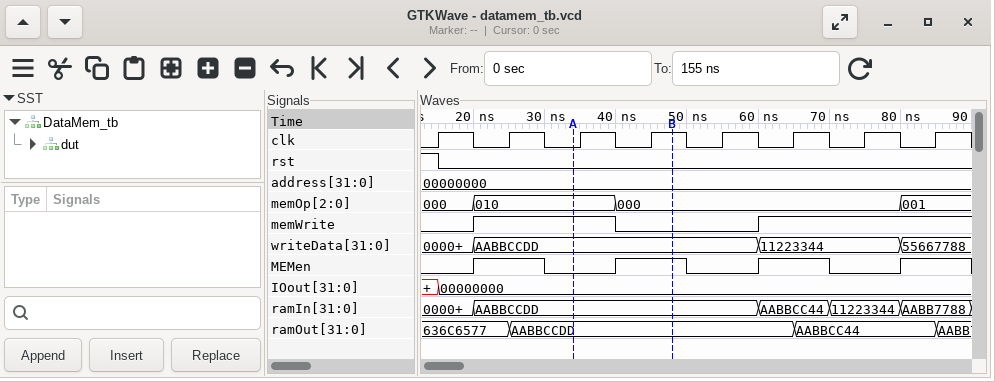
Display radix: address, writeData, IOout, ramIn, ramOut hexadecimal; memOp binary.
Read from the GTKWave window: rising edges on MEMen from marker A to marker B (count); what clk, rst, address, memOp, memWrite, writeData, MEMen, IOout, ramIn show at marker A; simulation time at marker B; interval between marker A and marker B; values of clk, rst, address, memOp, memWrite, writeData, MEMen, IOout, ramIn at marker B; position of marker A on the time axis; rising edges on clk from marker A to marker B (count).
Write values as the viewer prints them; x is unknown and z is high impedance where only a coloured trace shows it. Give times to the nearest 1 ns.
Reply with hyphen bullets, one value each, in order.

- 1
- clk=0, rst=0, address=00000000, memOp=010, memWrite=1, writeData=AABBCCDD, MEMen=0, IOout=00000000, ramIn=AABBCCDD
- 48 ns
- 14 ns
- clk=1, rst=0, address=00000000, memOp=000, memWrite=0, writeData=AABBCCDD, MEMen=1, IOout=00000000, ramIn=AABBCCDD
- 34 ns
- 2
